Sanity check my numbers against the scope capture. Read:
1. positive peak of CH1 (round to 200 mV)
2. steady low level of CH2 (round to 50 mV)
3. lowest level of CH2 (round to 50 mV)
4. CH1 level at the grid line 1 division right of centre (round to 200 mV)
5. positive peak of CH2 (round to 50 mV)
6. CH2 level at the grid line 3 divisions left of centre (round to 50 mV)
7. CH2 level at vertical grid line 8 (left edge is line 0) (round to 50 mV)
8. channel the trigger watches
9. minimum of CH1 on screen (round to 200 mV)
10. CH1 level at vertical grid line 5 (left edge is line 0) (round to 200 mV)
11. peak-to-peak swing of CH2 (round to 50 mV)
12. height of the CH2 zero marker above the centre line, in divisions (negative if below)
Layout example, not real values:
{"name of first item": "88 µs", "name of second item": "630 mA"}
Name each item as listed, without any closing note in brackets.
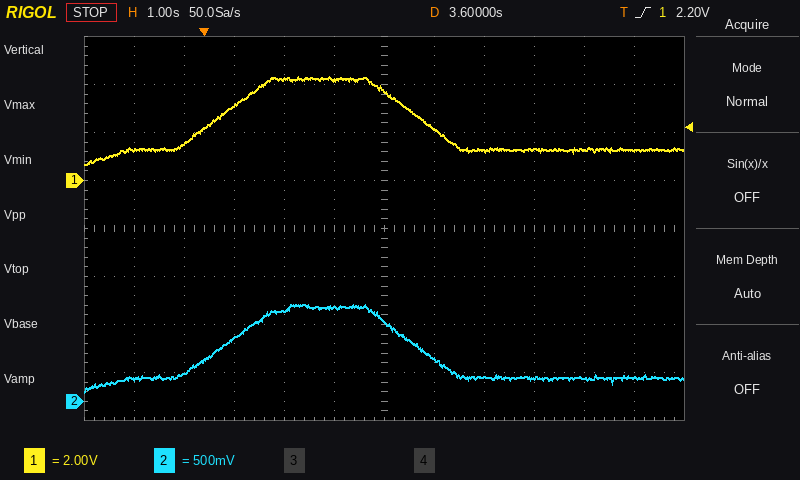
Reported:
{"positive peak of CH1": "4.4 V", "steady low level of CH2": "250 mV", "lowest level of CH2": "100 mV", "CH1 level at the grid line 1 division right of centre": "2.2 V", "positive peak of CH2": "1.00 V", "CH2 level at the grid line 3 divisions left of centre": "650 mV", "CH2 level at vertical grid line 8 (left edge is line 0)": "250 mV", "channel the trigger watches": "CH1", "minimum of CH1 on screen": "600 mV", "CH1 level at vertical grid line 5 (left edge is line 0)": "4.2 V", "peak-to-peak swing of CH2": "900 mV", "height of the CH2 zero marker above the centre line, in divisions": "-3.6 div"}
